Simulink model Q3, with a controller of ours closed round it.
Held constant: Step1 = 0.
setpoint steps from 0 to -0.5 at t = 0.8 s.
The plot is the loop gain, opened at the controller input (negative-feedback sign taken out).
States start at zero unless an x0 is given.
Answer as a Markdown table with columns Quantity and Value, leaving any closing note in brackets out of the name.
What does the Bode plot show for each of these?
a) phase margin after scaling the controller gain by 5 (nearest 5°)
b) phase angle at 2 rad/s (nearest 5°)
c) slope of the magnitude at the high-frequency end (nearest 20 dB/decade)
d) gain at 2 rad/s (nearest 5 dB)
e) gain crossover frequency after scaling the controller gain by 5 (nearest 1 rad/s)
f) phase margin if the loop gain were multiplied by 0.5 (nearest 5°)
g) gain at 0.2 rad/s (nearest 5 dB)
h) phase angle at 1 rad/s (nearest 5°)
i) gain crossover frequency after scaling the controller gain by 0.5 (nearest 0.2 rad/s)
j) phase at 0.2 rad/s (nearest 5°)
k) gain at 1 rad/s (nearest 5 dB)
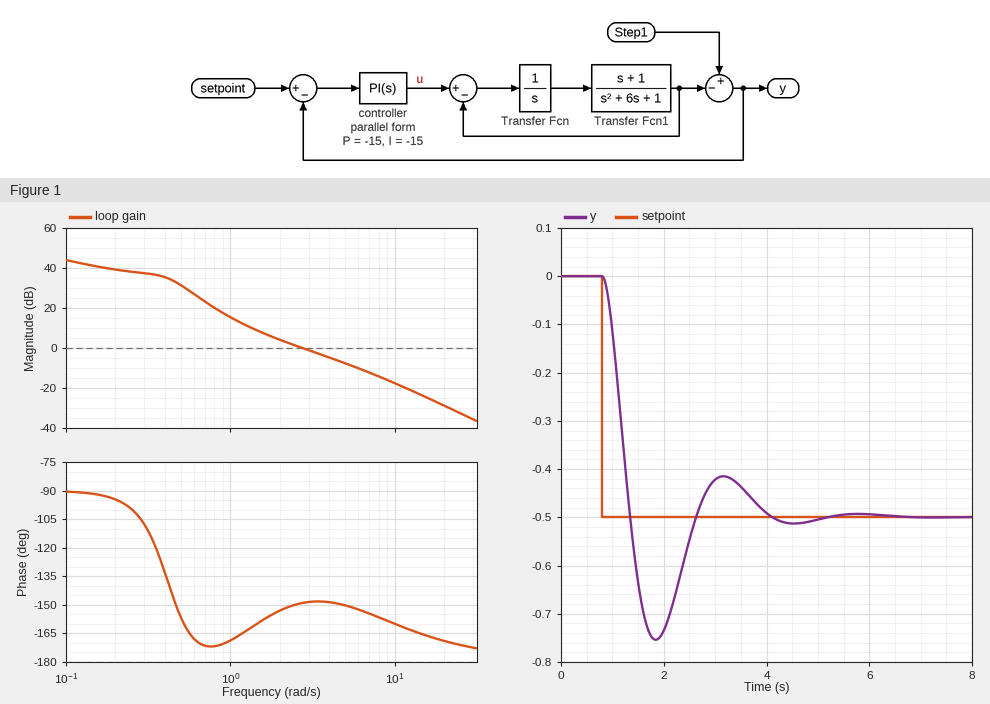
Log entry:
| Quantity | Value |
|---|---|
| phase margin after scaling the controller gain by 5 | 25° |
| phase angle at 2 rad/s | -155° |
| slope of the magnitude at the high-frequency end | -40 dB/decade |
| gain at 2 rad/s | 5 dB |
| gain crossover frequency after scaling the controller gain by 5 | 8 rad/s |
| phase margin if the loop gain were multiplied by 0.5 | 25° |
| gain at 0.2 rad/s | 40 dB |
| phase angle at 1 rad/s | -170° |
| gain crossover frequency after scaling the controller gain by 0.5 | 1.8 rad/s |
| phase at 0.2 rad/s | -95° |
| gain at 1 rad/s | 15 dB |
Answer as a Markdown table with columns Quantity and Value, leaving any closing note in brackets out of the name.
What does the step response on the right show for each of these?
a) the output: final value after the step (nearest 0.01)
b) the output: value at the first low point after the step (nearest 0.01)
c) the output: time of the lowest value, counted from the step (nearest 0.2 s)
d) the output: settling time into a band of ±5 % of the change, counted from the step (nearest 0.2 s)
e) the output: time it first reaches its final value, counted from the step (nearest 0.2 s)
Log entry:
| Quantity | Value |
|---|---|
| the output: final value after the step | -0.50 |
| the output: value at the first low point after the step | -0.75 |
| the output: time of the lowest value, counted from the step | 1.0 s |
| the output: settling time into a band of ±5 % of the change, counted from the step | 3.0 s |
| the output: time it first reaches its final value, counted from the step | 0.6 s |
